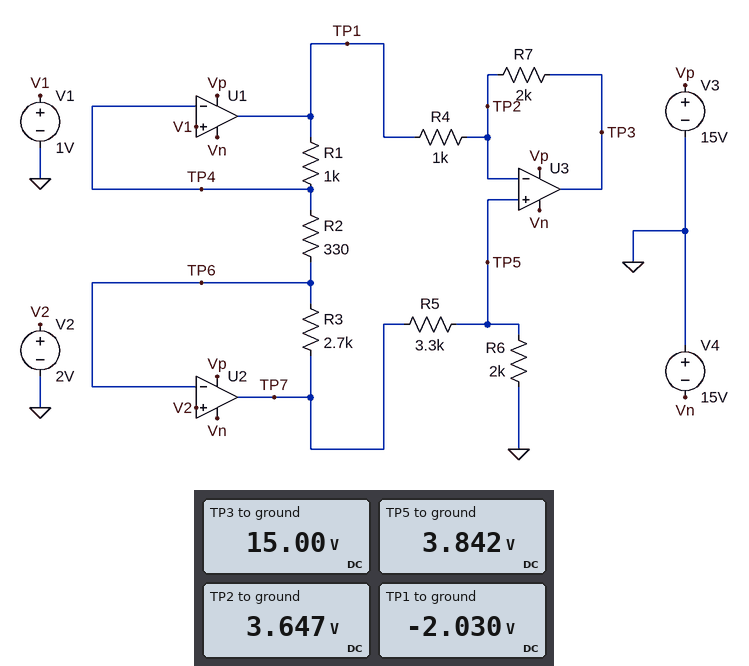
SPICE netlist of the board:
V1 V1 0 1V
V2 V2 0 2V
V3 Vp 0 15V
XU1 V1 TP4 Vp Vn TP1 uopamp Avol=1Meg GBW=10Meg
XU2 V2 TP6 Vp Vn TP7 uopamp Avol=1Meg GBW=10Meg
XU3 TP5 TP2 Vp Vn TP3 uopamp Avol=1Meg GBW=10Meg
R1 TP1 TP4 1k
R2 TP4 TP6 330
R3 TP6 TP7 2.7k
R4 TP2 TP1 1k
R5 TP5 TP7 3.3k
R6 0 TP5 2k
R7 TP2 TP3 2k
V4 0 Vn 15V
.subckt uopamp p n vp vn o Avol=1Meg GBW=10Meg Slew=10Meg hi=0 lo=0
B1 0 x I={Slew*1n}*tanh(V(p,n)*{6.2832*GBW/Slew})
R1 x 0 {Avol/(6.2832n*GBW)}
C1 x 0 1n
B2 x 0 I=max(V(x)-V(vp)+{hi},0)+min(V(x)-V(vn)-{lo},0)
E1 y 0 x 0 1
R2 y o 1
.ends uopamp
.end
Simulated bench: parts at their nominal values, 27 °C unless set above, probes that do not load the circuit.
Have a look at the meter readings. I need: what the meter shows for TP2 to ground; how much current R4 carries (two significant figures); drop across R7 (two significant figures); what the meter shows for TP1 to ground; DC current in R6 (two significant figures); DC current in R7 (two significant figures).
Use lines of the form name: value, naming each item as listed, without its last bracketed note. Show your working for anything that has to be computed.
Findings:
what the meter shows for TP2 to ground: 3.647 V
how much current R4 carries: (3.647 V - (-2.03 V)) / 1 kΩ = 5.7 mA
drop across R7: 15 V - 3.647 V = 11 V
what the meter shows for TP1 to ground: -2.030 V
DC current in R6: (3.842 V) / 2 kΩ = 1.9 mA
DC current in R7: (15 V - 3.647 V) / 2 kΩ = 5.7 mA
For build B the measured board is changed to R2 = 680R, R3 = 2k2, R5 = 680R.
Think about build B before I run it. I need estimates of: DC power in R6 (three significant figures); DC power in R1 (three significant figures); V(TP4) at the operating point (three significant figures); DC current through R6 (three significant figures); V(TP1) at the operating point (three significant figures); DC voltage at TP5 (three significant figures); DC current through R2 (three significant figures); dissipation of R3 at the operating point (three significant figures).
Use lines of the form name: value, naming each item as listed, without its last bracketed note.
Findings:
DC power in R6: 7.63 mW
DC power in R1: 2.16 mW
V(TP4) at the operating point: 1.00 V
DC current through R6: 1.95 mA
V(TP1) at the operating point: -471 mV
DC voltage at TP5: 3.91 V
DC current through R2: 1.47 mA
dissipation of R3 at the operating point: 4.76 mW
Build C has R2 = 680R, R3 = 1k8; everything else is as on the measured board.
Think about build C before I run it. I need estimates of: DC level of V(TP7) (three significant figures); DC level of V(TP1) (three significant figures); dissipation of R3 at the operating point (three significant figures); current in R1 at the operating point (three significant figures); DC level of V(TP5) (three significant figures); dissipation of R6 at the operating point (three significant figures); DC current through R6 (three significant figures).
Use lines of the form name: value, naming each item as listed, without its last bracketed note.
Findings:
DC level of V(TP7): 4.65 V
DC level of V(TP1): -471 mV
dissipation of R3 at the operating point: 3.89 mW
current in R1 at the operating point: 1.47 mA
DC level of V(TP5): 1.75 V
dissipation of R6 at the operating point: 1.54 mW
DC current through R6: 877 µA
